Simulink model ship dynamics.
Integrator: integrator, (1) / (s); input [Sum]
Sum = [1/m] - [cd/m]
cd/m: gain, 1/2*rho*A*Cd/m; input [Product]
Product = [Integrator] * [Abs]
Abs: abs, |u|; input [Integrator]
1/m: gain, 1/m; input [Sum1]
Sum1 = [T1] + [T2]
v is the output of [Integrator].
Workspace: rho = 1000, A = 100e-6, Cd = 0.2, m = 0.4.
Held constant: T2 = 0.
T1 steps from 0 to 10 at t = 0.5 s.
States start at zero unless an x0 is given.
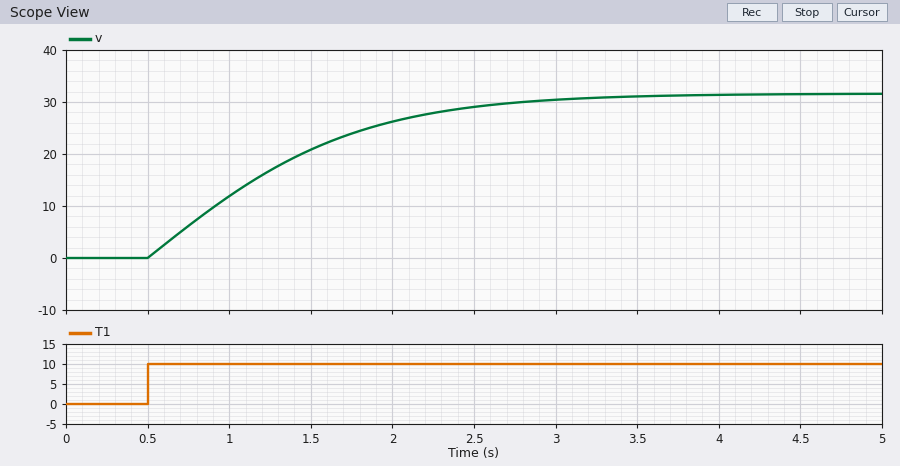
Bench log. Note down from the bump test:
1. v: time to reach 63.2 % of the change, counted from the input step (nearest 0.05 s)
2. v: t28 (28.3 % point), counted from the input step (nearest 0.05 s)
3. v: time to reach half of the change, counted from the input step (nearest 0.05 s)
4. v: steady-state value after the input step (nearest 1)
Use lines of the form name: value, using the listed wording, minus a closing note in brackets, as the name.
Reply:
v: time to reach 63.2 % of the change, counted from the input step: 0.95 s
v: t28 (28.3 % point), counted from the input step: 0.35 s
v: time to reach half of the change, counted from the input step: 0.70 s
v: steady-state value after the input step: 32
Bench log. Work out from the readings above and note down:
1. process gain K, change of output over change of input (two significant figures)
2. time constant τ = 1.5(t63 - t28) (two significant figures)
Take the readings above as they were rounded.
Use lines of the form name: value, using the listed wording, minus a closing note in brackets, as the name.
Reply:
process gain K, change of output over change of input: 3.2
time constant τ = 1.5(t63 - t28): 0.90 s
